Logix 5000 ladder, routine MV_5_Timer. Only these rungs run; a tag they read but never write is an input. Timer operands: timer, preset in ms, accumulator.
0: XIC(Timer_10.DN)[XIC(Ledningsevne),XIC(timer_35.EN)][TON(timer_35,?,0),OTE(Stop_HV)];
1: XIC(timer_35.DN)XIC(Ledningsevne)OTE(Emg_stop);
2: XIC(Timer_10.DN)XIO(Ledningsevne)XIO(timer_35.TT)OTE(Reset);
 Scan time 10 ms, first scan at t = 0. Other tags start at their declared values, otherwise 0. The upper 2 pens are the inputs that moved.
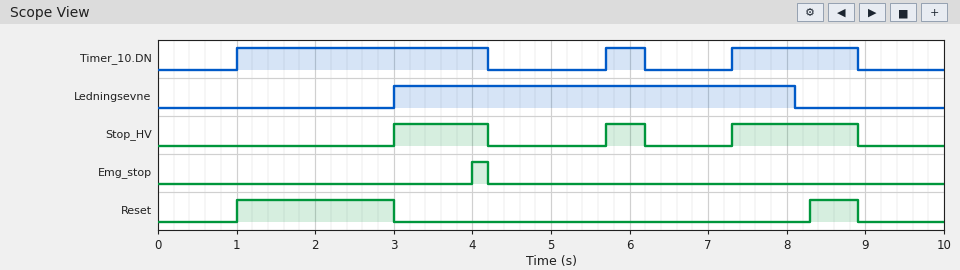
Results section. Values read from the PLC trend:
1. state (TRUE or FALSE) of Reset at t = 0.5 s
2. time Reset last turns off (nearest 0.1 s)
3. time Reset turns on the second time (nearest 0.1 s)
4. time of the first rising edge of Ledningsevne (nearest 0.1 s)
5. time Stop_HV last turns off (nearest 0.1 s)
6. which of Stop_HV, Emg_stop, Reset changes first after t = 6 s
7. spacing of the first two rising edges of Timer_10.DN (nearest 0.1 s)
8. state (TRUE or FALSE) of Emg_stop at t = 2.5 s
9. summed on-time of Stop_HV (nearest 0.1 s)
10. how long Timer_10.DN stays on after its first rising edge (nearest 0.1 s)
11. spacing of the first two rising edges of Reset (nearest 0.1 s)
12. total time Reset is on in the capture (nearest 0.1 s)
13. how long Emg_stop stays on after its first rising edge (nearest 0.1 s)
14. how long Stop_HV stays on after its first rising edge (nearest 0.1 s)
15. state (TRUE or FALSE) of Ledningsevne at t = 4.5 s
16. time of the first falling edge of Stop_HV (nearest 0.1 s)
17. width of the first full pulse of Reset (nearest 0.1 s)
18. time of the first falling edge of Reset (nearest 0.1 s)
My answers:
FALSE
8.9 s
8.3 s
3.0 s
8.9 s
Stop_HV
4.7 s
FALSE
3.3 s
3.2 s
7.3 s
2.6 s
0.2 s
1.2 s
TRUE
4.2 s
2.0 s
3.0 s
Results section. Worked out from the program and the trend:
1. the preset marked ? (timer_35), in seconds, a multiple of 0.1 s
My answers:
1.0 s
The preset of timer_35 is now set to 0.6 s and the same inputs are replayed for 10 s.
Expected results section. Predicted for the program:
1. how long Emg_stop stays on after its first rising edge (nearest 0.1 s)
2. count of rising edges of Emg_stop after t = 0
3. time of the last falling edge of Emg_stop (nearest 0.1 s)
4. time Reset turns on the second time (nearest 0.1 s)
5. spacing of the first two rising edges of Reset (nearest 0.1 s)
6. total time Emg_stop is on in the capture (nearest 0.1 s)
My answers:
0.6 s
2
8.1 s
8.1 s
7.1 s
0.8 s
